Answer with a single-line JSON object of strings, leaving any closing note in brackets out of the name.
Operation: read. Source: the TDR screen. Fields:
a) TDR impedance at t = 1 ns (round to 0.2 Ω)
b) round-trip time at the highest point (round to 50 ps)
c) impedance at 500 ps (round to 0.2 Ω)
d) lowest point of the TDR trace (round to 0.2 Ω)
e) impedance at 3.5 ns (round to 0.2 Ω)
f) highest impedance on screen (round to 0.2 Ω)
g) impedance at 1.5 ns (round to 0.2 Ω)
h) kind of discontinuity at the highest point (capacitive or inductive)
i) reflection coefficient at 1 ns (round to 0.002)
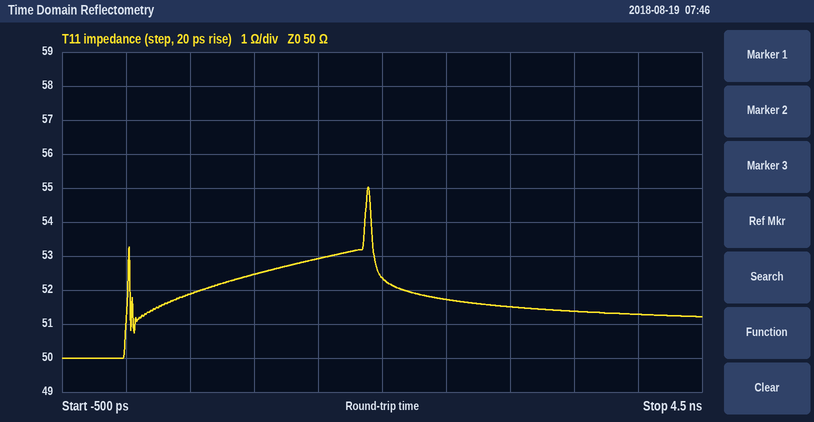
{"TDR impedance at t = 1 ns": "52.4 Ω", "round-trip time at the highest point": "1.90 ns", "impedance at 500 ps": "51.8 Ω", "lowest point of the TDR trace": "50.0 Ω", "impedance at 3.5 ns": "51.4 Ω", "highest impedance on screen": "55.0 Ω", "impedance at 1.5 ns": "53.0 Ω", "kind of discontinuity at the highest point": "inductive", "reflection coefficient at 1 ns": "+0.024"}
